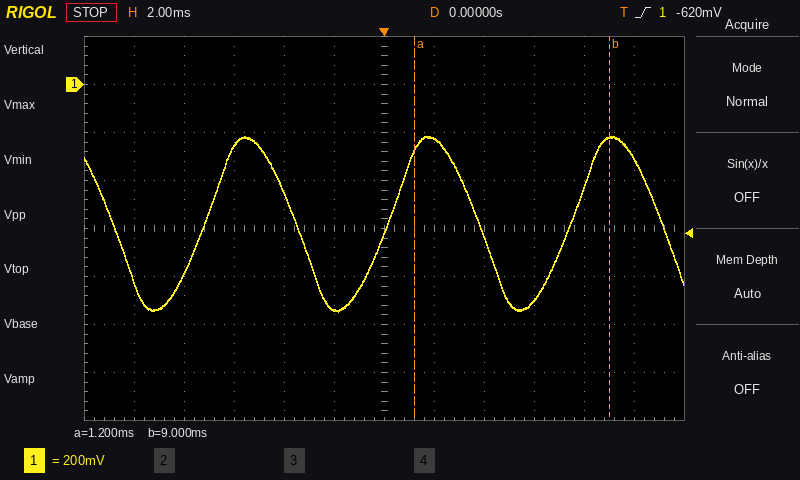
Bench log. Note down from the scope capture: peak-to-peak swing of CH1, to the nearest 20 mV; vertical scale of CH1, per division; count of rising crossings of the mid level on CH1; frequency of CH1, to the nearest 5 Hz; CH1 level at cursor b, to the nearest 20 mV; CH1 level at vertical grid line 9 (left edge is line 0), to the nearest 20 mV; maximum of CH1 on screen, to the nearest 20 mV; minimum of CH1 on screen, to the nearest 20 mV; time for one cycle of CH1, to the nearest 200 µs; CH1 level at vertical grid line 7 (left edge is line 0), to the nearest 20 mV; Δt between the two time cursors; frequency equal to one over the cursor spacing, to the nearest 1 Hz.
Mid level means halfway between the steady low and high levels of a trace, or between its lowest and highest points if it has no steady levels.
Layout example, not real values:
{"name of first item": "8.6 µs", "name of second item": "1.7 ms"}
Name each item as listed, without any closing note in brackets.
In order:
{"peak-to-peak swing of CH1, to the nearest 20 mV": "720 mV", "vertical scale of CH1, per division": "200 mV", "count of rising crossings of the mid level on CH1": "3", "frequency of CH1, to the nearest 5 Hz": "135 Hz", "CH1 level at cursor b, to the nearest 20 mV": "-220 mV", "CH1 level at vertical grid line 9 (left edge is line 0), to the nearest 20 mV": "-900 mV", "maximum of CH1 on screen, to the nearest 20 mV": "-220 mV", "minimum of CH1 on screen, to the nearest 20 mV": "-940 mV", "time for one cycle of CH1, to the nearest 200 µs": "7.4 ms", "CH1 level at vertical grid line 7 (left edge is line 0), to the nearest 20 mV": "-220 mV", "Δt between the two time cursors": "7.8 ms", "frequency equal to one over the cursor spacing, to the nearest 1 Hz": "128 Hz"}
